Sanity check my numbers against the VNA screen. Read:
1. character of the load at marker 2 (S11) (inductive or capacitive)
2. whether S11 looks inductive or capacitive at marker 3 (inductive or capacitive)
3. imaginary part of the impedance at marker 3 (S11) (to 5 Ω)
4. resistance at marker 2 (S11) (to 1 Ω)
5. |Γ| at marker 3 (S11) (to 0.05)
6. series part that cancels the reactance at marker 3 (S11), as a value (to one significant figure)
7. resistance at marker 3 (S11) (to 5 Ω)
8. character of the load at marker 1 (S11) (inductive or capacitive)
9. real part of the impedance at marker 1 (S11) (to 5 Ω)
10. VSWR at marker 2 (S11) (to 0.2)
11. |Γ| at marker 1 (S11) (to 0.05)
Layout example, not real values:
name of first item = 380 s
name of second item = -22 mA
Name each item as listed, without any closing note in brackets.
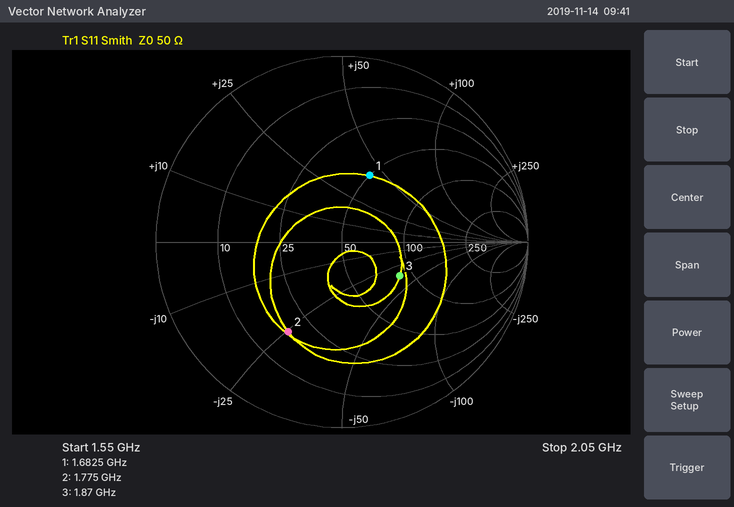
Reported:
character of the load at marker 2 (S11) = capacitive
whether S11 looks inductive or capacitive at marker 3 = capacitive
imaginary part of the impedance at marker 3 (S11) = -35 Ω
resistance at marker 2 (S11) = 18 Ω
|Γ| at marker 3 (S11) = 0.35
series part that cancels the reactance at marker 3 (S11), as a value = 3 nH
resistance at marker 3 (S11) = 85 Ω
character of the load at marker 1 (S11) = inductive
real part of the impedance at marker 1 (S11) = 50 Ω
VSWR at marker 2 (S11) = 3.6
|Γ| at marker 1 (S11) = 0.40
